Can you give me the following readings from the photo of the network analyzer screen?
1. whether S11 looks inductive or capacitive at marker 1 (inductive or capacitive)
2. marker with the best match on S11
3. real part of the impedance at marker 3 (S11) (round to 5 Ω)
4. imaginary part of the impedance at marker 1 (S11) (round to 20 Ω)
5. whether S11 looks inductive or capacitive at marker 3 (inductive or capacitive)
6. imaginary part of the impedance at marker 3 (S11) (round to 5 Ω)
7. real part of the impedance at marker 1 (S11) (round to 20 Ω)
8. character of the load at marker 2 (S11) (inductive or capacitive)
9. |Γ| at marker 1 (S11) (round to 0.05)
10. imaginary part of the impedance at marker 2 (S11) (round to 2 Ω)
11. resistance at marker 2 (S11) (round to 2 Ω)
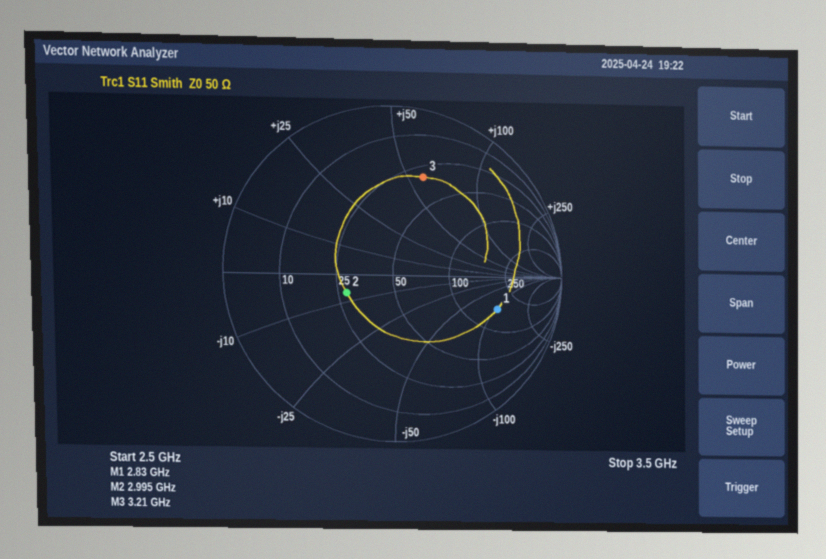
capacitive
marker 2
30 Ω
-100 Ω
inductive
+60 Ω
160 Ω
capacitive
0.65
-6 Ω
28 Ω
